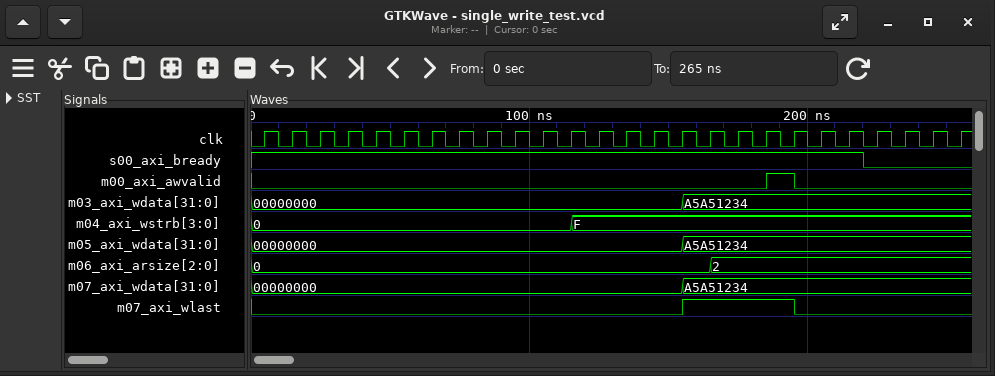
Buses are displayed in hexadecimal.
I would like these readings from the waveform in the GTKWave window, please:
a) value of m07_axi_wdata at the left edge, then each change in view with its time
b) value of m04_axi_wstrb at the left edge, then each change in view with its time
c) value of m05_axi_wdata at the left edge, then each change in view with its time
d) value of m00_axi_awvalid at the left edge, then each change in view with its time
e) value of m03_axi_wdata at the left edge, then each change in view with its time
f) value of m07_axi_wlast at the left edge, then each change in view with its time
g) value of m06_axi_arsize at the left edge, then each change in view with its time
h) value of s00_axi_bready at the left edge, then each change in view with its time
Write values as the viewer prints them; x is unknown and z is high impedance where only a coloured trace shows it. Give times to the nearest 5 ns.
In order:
00000000, A5A51234 at 155 ns
0, F at 115 ns
00000000, A5A51234 at 155 ns
0, 1 at 185 ns, 0 at 195 ns
00000000, A5A51234 at 155 ns
0, 1 at 155 ns, 0 at 195 ns
0, 2 at 165 ns
1, 0 at 220 ns
